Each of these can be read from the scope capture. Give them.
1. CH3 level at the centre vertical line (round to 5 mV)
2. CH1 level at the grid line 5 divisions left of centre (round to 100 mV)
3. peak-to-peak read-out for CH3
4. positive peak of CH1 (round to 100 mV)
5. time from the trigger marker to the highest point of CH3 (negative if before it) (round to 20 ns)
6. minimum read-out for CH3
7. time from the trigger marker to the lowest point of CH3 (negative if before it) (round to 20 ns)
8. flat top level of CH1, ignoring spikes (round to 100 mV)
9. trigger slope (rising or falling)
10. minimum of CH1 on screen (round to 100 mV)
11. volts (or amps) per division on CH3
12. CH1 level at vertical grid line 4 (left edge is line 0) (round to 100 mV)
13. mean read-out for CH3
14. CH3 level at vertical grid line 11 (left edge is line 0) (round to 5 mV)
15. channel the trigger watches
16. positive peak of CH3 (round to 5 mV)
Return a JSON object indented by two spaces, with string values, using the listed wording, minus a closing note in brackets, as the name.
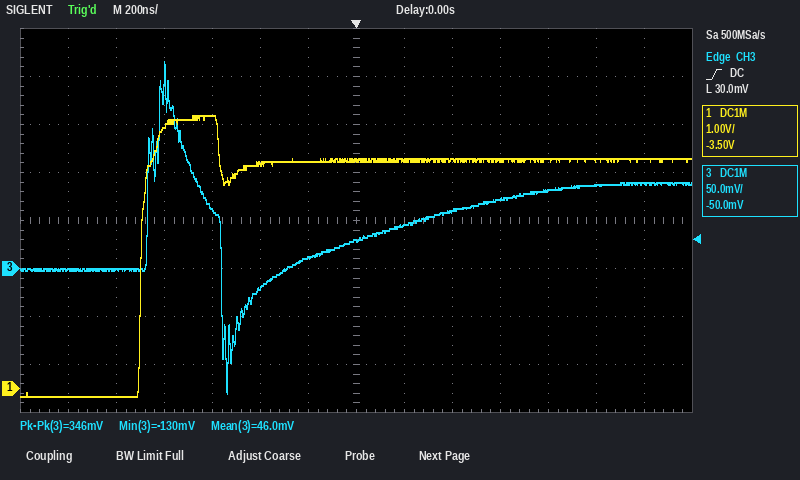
{
  "CH3 level at the centre vertical line": "30 mV",
  "CH1 level at the grid line 5 divisions left of centre": "-200 mV",
  "peak-to-peak read-out for CH3": "346 mV",
  "positive peak of CH1": "5.7 V",
  "time from the trigger marker to the highest point of CH3 (negative if before it)": "-800 ns",
  "minimum read-out for CH3": "-130 mV",
  "time from the trigger marker to the lowest point of CH3 (negative if before it)": "-540 ns",
  "flat top level of CH1, ignoring spikes": "4.8 V",
  "trigger slope": "rising",
  "minimum of CH1 on screen": "-200 mV",
  "volts (or amps) per division on CH3": "50 mV",
  "CH1 level at vertical grid line 4 (left edge is line 0)": "5.7 V",
  "mean read-out for CH3": "46.0 mV",
  "CH3 level at vertical grid line 11 (left edge is line 0)": "80 mV",
  "channel the trigger watches": "CH3",
  "positive peak of CH3": "215 mV"
}
